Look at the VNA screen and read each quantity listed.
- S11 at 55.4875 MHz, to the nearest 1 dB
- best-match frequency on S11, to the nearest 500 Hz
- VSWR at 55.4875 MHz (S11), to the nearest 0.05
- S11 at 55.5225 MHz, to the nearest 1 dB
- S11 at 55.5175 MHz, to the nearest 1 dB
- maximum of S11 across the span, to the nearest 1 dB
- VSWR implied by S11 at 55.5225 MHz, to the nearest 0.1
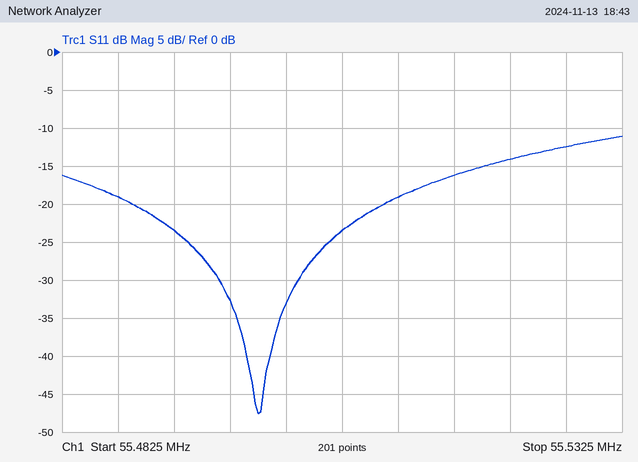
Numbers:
-19 dB
55.5000 MHz
1.25
-14 dB
-16 dB
-11 dB
1.5
